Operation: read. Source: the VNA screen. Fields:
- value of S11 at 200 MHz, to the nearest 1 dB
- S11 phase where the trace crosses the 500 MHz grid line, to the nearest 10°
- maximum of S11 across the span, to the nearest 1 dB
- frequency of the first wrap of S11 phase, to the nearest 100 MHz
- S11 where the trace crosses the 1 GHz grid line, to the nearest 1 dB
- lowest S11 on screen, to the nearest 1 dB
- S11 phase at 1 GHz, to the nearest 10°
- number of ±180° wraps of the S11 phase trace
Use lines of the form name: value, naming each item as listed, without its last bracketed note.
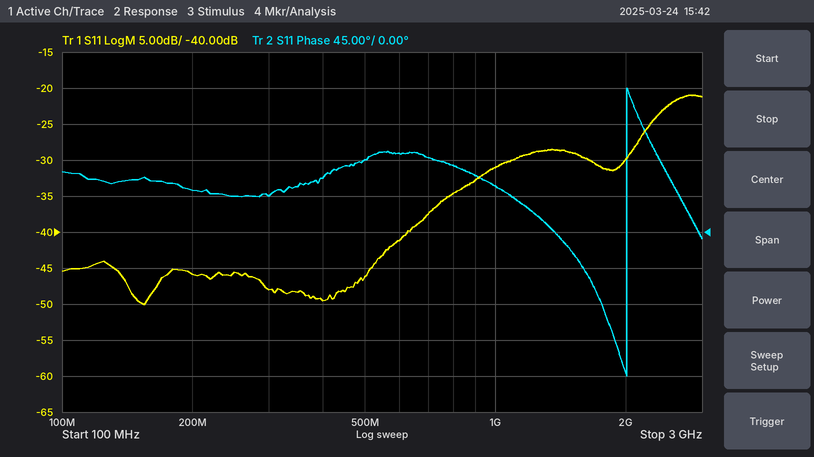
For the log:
value of S11 at 200 MHz, to the nearest 1 dB: -46 dB
S11 phase where the trace crosses the 500 MHz grid line, to the nearest 10°: 90°
maximum of S11 across the span, to the nearest 1 dB: -21 dB
frequency of the first wrap of S11 phase, to the nearest 100 MHz: 2.0 GHz
S11 where the trace crosses the 1 GHz grid line, to the nearest 1 dB: -31 dB
lowest S11 on screen, to the nearest 1 dB: -50 dB
S11 phase at 1 GHz, to the nearest 10°: 60°
number of ±180° wraps of the S11 phase trace: 1
